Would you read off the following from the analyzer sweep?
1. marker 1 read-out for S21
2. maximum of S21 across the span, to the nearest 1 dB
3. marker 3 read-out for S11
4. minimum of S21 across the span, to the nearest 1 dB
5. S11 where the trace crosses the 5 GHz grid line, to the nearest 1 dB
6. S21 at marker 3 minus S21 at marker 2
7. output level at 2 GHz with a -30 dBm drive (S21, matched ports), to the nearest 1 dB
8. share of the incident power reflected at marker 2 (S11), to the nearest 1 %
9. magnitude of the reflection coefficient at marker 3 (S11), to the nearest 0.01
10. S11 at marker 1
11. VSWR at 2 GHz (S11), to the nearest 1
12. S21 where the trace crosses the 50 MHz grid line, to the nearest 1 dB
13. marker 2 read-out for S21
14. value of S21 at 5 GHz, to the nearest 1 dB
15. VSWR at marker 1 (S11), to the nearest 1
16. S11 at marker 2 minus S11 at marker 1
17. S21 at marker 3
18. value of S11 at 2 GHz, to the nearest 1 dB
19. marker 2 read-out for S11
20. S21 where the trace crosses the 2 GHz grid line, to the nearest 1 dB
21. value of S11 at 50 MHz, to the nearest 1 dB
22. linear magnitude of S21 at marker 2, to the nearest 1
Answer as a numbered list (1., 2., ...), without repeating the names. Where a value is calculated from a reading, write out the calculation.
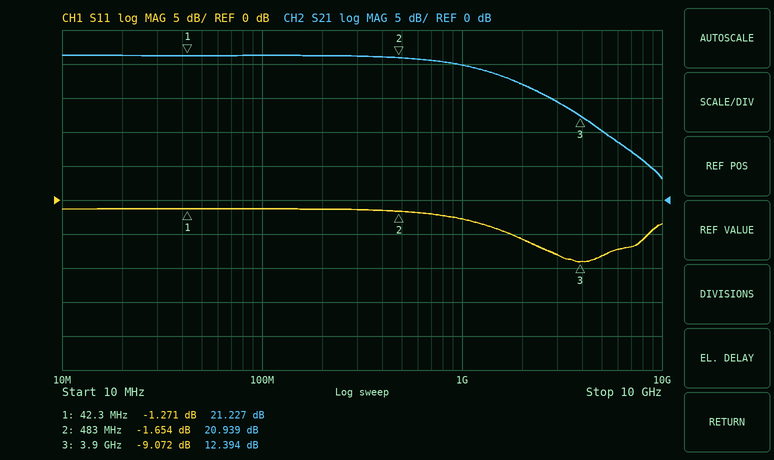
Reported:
1. 21.227 dB
2. 21 dB
3. -9.072 dB
4. 3 dB
5. -8 dB
6. 12.394 − (20.939) = -8.545 dB
7. -30 dBm + (17 dB) = -13 dBm
8. 10^(-1.654/10) ≈ 68 %
9. 10^(-9.072/20) ≈ 0.35
10. -1.271 dB
11. |Γ| = 10^(-6/20) = 0.5012; VSWR = (1 + 0.5012)/(1 − 0.5012) ≈ 3
12. 21 dB
13. 20.939 dB
14. 10 dB
15. (1 + 0.8639)/(1 − 0.8639) ≈ 14
16. -1.654 − (-1.271) = -0.383 dB
17. 12.394 dB
18. -6 dB
19. -1.654 dB
20. 17 dB
21. -1 dB
22. 10^(20.939/20) ≈ 11
